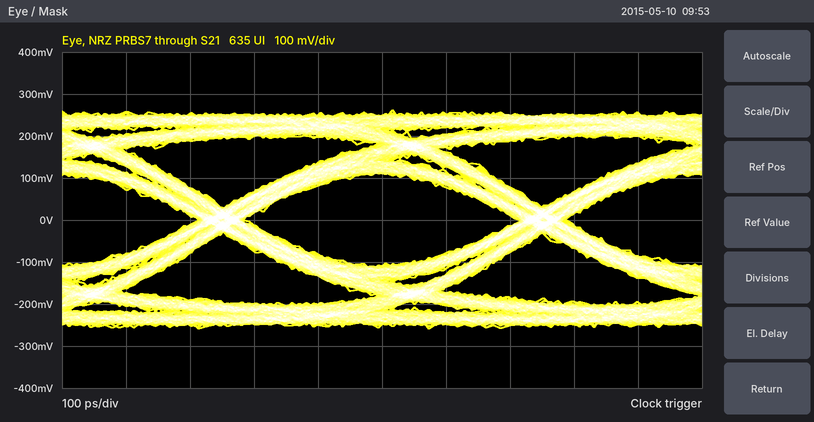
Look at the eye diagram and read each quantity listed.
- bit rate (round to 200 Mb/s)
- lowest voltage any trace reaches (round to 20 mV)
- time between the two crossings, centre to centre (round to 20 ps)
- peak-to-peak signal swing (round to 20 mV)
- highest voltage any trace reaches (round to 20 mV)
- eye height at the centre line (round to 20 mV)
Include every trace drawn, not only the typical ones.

2.0 Gb/s
-260 mV
500 ps
520 mV
260 mV
220 mV
